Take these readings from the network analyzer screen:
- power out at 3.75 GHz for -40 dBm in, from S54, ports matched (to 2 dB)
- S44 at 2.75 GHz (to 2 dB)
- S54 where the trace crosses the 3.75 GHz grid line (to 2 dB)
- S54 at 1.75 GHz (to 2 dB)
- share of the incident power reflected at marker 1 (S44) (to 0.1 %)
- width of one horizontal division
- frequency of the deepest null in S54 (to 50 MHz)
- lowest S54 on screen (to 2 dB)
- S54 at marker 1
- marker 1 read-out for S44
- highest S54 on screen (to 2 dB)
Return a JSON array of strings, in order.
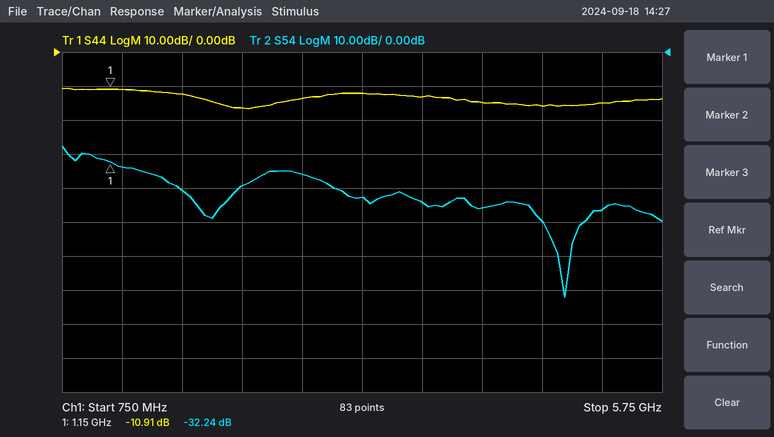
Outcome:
["-84 dBm", "-14 dB", "-44 dB", "-40 dB", "8.1 %", "500 MHz", "4.95 GHz", "-72 dB", "-32.24 dB", "-10.91 dB", "-28 dB"]
